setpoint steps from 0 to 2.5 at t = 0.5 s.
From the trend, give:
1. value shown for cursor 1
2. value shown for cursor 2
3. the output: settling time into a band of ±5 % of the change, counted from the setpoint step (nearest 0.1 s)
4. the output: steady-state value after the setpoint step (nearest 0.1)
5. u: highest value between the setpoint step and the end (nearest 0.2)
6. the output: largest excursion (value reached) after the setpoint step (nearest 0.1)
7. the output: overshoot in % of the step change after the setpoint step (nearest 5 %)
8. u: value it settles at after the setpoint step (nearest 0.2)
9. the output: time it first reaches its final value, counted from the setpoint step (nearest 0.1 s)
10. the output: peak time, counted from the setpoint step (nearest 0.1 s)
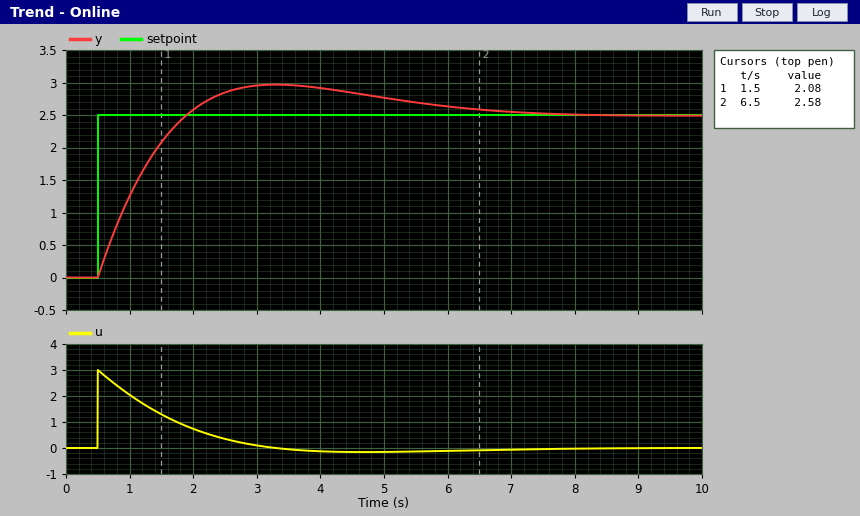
2.08
2.58
5.6 s
2.5
3.0
3.0
20 %
0.0
1.4 s
2.8 s
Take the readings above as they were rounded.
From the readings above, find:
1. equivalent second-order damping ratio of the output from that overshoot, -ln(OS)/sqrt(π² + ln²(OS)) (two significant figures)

0.46
